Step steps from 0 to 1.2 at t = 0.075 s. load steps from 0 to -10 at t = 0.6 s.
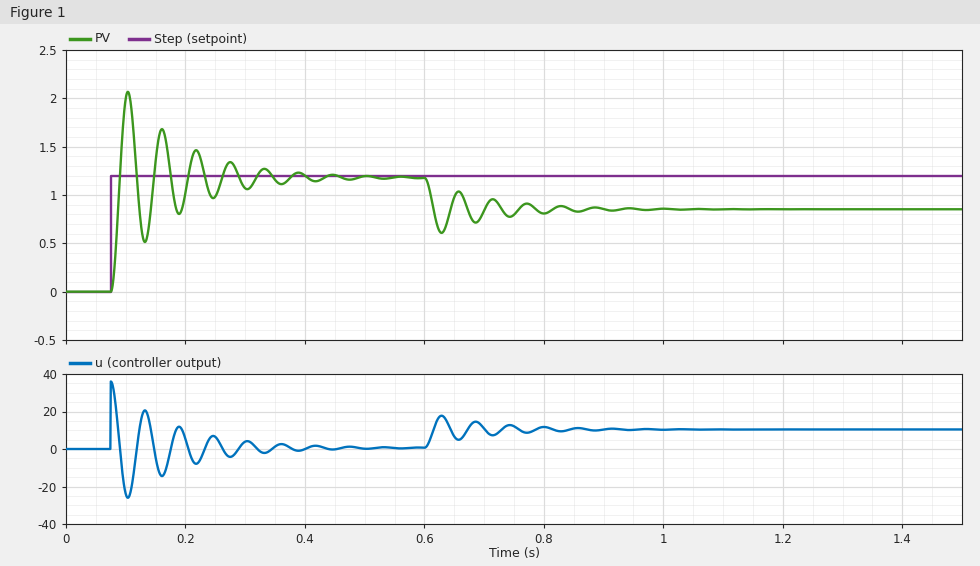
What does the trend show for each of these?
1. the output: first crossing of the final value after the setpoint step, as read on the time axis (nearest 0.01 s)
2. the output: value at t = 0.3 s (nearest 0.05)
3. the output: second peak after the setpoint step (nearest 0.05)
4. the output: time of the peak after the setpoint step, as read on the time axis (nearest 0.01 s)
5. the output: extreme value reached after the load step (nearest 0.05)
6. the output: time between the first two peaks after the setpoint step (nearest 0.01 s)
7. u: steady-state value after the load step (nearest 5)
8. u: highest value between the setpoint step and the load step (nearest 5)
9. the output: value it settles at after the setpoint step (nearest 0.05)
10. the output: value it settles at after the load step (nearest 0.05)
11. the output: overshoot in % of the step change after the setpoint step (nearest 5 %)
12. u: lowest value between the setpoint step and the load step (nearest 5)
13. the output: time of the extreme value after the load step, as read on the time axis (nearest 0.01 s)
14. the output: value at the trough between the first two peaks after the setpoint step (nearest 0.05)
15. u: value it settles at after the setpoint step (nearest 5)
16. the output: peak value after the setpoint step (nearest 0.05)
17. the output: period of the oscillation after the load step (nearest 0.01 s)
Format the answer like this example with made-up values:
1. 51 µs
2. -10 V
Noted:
1. 0.09 s
2. 1.05
3. 1.70
4. 0.10 s
5. 0.60
6. 0.06 s
7. 10
8. 35
9. 1.20
10. 0.85
11. 75 %
12. -25
13. 0.63 s
14. 0.50
15. 0
16. 2.05
17. 0.06 s
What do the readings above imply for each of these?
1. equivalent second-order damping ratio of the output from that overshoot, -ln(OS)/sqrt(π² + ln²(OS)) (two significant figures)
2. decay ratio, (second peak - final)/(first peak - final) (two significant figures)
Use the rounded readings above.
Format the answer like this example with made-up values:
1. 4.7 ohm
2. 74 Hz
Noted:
1. 0.091
2. 0.59
